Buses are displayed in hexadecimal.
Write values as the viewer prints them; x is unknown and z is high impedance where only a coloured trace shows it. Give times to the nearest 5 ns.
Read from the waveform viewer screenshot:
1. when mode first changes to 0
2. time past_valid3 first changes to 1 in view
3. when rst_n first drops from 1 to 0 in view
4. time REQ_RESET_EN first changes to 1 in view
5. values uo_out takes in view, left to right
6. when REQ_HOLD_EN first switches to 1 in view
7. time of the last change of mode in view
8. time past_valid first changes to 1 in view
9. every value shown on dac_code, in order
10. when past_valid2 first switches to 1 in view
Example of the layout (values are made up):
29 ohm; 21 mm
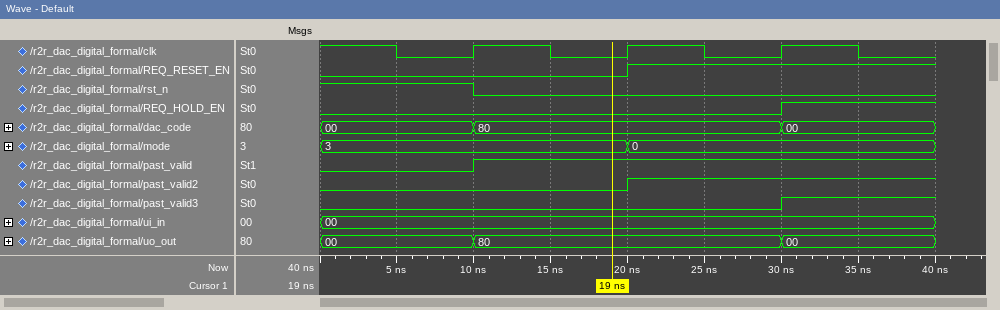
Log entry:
20 ns; 30 ns; 10 ns; 20 ns; 00, 80, 00; 30 ns; 20 ns; 10 ns; 00, 80, 00; 20 ns
